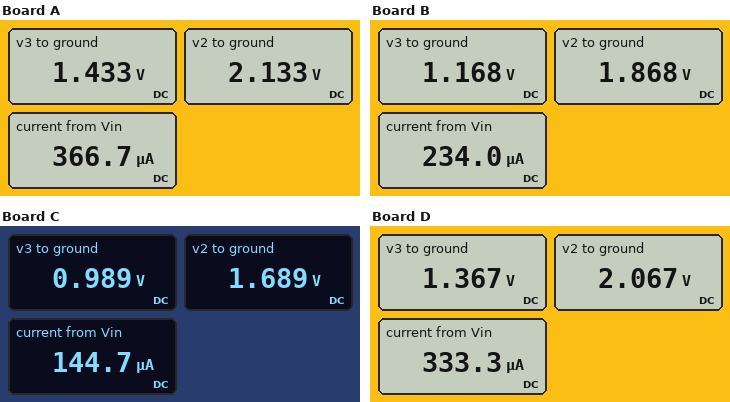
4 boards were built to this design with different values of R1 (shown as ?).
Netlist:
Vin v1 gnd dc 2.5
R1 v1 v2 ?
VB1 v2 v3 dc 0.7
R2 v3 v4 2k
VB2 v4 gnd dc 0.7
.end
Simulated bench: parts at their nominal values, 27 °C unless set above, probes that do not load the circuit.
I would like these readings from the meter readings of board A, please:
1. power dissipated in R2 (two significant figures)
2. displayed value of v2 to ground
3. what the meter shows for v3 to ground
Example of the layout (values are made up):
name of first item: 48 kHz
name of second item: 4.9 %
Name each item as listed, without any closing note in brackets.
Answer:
power dissipated in R2: 270 µW
displayed value of v2 to ground: 2.133 V
what the meter shows for v3 to ground: 1.433 V
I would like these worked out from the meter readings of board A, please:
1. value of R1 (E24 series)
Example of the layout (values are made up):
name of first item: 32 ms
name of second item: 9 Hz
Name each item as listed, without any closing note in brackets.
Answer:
value of R1: 1 kΩ
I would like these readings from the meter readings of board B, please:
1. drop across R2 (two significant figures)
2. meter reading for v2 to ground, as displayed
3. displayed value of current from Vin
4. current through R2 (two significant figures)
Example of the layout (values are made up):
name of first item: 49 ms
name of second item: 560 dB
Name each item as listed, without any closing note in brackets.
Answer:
drop across R2: 470 mV
meter reading for v2 to ground, as displayed: 1.868 V
displayed value of current from Vin: 234.0 µA
current through R2: 230 µA
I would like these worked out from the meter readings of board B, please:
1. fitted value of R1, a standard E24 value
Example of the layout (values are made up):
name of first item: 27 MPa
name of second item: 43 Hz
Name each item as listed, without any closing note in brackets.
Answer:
fitted value of R1, a standard E24 value: 2.7 kΩ
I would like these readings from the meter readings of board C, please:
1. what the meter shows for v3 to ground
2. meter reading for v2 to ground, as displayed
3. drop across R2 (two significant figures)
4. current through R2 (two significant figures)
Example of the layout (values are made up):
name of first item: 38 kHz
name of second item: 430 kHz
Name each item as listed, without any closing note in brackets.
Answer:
what the meter shows for v3 to ground: 0.989 V
meter reading for v2 to ground, as displayed: 1.689 V
drop across R2: 290 mV
current through R2: 140 µA
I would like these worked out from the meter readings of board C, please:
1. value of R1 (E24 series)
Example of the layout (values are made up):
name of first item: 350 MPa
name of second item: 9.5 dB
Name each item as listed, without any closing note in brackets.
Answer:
value of R1: 5.6 kΩ
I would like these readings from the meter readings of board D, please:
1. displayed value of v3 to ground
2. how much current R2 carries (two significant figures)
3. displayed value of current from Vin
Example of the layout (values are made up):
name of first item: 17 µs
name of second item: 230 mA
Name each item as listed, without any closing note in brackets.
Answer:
displayed value of v3 to ground: 1.367 V
how much current R2 carries: 330 µA
displayed value of current from Vin: 333.3 µA
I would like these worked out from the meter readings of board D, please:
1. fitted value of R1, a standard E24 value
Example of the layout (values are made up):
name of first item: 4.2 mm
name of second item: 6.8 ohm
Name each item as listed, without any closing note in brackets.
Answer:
fitted value of R1, a standard E24 value: 1.3 kΩ
